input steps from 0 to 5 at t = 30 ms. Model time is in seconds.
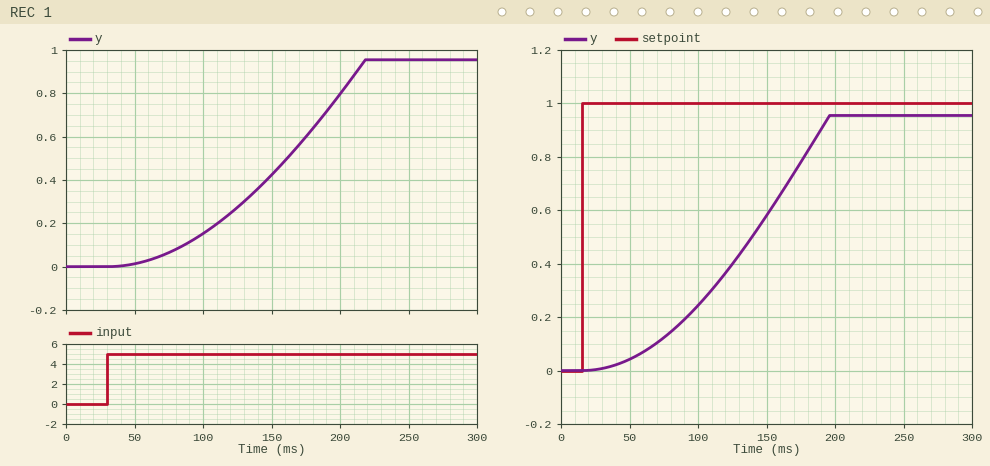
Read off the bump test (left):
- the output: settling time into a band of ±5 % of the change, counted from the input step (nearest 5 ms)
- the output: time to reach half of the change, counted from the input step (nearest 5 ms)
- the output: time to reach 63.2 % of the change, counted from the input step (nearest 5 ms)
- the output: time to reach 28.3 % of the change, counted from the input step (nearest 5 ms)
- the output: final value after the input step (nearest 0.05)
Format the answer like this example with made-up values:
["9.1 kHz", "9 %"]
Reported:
["185 ms", "130 ms", "145 ms", "95 ms", "0.95"]
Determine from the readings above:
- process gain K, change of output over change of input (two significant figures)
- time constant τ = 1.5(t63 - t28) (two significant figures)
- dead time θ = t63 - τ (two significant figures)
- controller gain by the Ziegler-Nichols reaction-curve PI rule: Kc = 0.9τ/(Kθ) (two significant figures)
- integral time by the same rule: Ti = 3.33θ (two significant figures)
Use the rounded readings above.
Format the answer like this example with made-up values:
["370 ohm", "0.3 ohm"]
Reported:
["0.19", "75 ms", "70 ms", "5.1", "230 ms"]
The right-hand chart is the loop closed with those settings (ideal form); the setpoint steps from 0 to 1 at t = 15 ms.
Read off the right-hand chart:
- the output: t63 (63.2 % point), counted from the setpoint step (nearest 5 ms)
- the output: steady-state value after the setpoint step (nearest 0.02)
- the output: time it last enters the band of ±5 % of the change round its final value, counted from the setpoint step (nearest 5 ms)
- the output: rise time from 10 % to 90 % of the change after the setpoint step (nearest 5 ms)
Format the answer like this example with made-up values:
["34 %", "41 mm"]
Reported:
["140 ms", "0.96", "175 ms", "115 ms"]
